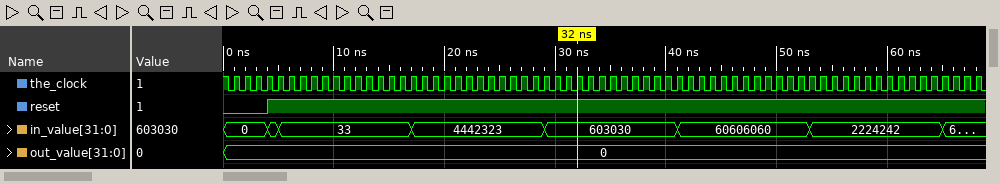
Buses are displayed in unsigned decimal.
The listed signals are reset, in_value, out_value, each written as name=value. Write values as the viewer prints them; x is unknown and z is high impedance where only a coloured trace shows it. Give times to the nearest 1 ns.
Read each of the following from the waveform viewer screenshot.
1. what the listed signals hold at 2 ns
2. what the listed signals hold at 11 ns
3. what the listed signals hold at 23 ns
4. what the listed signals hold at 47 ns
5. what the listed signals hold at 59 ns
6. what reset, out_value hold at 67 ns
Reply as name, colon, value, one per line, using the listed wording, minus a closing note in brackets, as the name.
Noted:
what the listed signals hold at 2 ns: reset=0, in_value=0, out_value=0
what the listed signals hold at 11 ns: reset=1, in_value=33, out_value=0
what the listed signals hold at 23 ns: reset=1, in_value=4442323, out_value=0
what the listed signals hold at 47 ns: reset=1, in_value=60606060, out_value=0
what the listed signals hold at 59 ns: reset=1, in_value=2224242, out_value=0
what reset, out_value hold at 67 ns: reset=1, out_value=0
